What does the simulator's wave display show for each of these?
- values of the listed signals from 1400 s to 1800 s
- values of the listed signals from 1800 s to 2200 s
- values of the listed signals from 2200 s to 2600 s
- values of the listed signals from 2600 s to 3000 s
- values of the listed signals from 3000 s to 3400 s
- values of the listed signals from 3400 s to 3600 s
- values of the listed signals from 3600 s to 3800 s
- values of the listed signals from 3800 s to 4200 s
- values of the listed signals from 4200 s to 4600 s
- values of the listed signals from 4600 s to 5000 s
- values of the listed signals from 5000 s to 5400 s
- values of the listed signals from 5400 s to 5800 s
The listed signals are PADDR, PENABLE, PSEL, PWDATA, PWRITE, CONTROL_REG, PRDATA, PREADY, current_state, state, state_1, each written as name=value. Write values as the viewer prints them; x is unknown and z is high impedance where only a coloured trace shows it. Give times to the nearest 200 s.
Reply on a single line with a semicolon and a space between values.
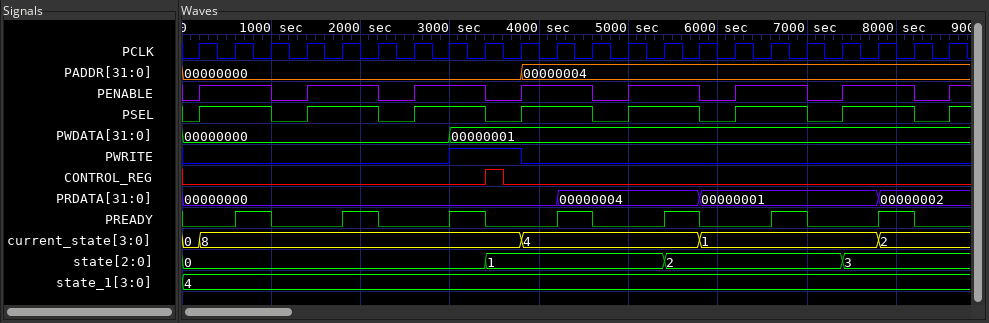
PADDR=00000000, PENABLE=1, PSEL=1, PWDATA=00000000, PWRITE=0, CONTROL_REG=0, PRDATA=00000000, PREADY=0, current_state=8, state=0, state_1=4; PADDR=00000000, PENABLE=1, PSEL=1, PWDATA=00000000, PWRITE=0, CONTROL_REG=0, PRDATA=00000000, PREADY=1, current_state=8, state=0, state_1=4; PADDR=00000000, PENABLE=0, PSEL=0, PWDATA=00000000, PWRITE=0, CONTROL_REG=0, PRDATA=00000000, PREADY=0, current_state=8, state=0, state_1=4; PADDR=00000000, PENABLE=1, PSEL=1, PWDATA=00000000, PWRITE=0, CONTROL_REG=0, PRDATA=00000000, PREADY=0, current_state=8, state=0, state_1=4; PADDR=00000000, PENABLE=1, PSEL=1, PWDATA=00000001, PWRITE=1, CONTROL_REG=0, PRDATA=00000000, PREADY=1, current_state=8, state=0, state_1=4; PADDR=00000000, PENABLE=0, PSEL=0, PWDATA=00000001, PWRITE=1, CONTROL_REG=1, PRDATA=00000000, PREADY=0, current_state=8, state=1, state_1=4; PADDR=00000000, PENABLE=0, PSEL=0, PWDATA=00000001, PWRITE=1, CONTROL_REG=0, PRDATA=00000000, PREADY=0, current_state=8, state=1, state_1=4; PADDR=00000004, PENABLE=1, PSEL=1, PWDATA=00000001, PWRITE=0, CONTROL_REG=0, PRDATA=00000000, PREADY=0, current_state=4, state=1, state_1=4; PADDR=00000004, PENABLE=1, PSEL=1, PWDATA=00000001, PWRITE=0, CONTROL_REG=0, PRDATA=00000004, PREADY=1, current_state=4, state=1, state_1=4; PADDR=00000004, PENABLE=0, PSEL=0, PWDATA=00000001, PWRITE=0, CONTROL_REG=0, PRDATA=00000004, PREADY=0, current_state=4, state=1, state_1=4; PADDR=00000004, PENABLE=1, PSEL=1, PWDATA=00000001, PWRITE=0, CONTROL_REG=0, PRDATA=00000004, PREADY=0, current_state=4, state=1, state_1=4; PADDR=00000004, PENABLE=1, PSEL=1, PWDATA=00000001, PWRITE=0, CONTROL_REG=0, PRDATA=00000004, PREADY=1, current_state=4, state=2, state_1=4
